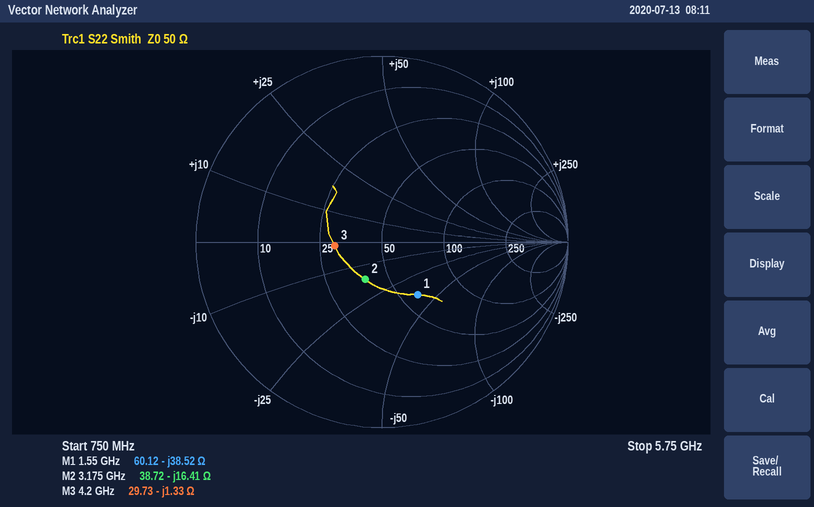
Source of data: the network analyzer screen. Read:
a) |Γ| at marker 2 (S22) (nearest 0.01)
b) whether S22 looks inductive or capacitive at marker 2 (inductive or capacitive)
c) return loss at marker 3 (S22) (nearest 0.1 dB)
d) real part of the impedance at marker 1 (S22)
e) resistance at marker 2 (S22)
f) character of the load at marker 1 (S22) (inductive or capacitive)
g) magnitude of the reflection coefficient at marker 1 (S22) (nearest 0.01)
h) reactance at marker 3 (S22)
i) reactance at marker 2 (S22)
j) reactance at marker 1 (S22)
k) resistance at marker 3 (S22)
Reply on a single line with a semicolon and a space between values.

0.22; capacitive; 11.9 dB; 60.12 Ω; 38.72 Ω; capacitive; 0.34; -1.33 Ω; -16.41 Ω; -38.52 Ω; 29.73 Ω
